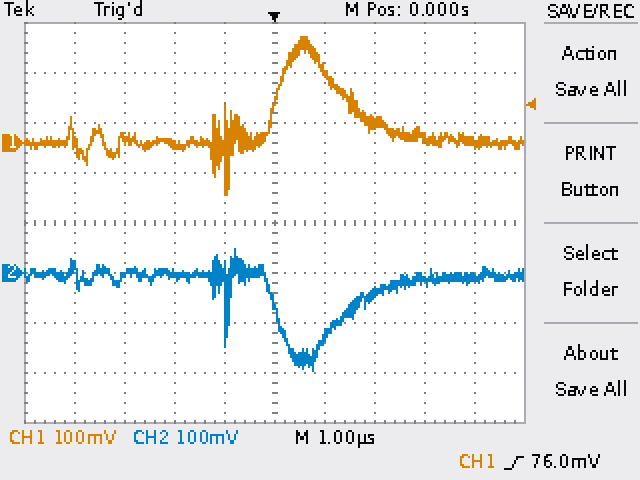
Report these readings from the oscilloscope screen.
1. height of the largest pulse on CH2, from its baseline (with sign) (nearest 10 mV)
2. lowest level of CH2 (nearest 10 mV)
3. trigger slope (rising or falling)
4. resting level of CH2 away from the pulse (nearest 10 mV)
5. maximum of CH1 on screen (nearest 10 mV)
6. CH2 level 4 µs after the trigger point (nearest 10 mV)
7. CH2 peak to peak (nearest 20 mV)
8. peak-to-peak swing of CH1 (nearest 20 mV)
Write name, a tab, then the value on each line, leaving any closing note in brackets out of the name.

height of the largest pulse on CH2, from its baseline (with sign)	-190 mV
lowest level of CH2	-200 mV
trigger slope	rising
resting level of CH2 away from the pulse	-10 mV
maximum of CH1 on screen	210 mV
CH2 level 4 µs after the trigger point	-10 mV
CH2 peak to peak	240 mV
peak-to-peak swing of CH1	320 mV
